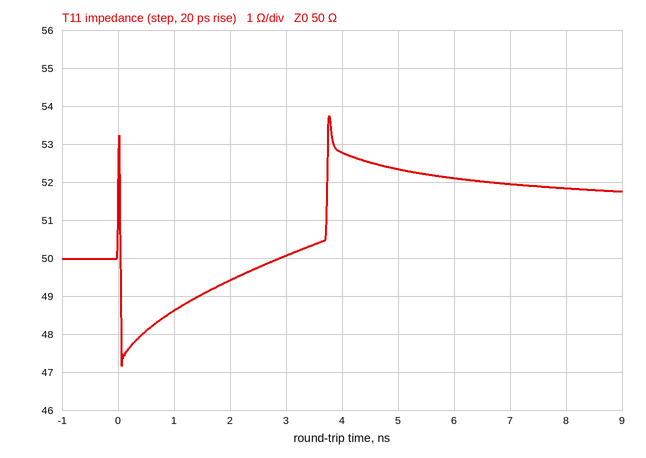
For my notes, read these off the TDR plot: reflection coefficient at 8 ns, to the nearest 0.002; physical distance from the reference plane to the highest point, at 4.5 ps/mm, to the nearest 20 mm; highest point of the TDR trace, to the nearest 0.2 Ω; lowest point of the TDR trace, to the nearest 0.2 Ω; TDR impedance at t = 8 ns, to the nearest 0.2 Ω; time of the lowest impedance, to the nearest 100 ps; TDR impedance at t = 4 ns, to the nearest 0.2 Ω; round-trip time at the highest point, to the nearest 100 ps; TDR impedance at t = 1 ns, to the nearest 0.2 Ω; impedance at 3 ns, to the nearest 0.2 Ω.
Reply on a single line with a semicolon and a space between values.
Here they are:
+0.018; 420 mm; 53.8 Ω; 47.2 Ω; 51.8 Ω; 100 ps; 52.8 Ω; 3.8 ns; 48.6 Ω; 50.0 Ω
